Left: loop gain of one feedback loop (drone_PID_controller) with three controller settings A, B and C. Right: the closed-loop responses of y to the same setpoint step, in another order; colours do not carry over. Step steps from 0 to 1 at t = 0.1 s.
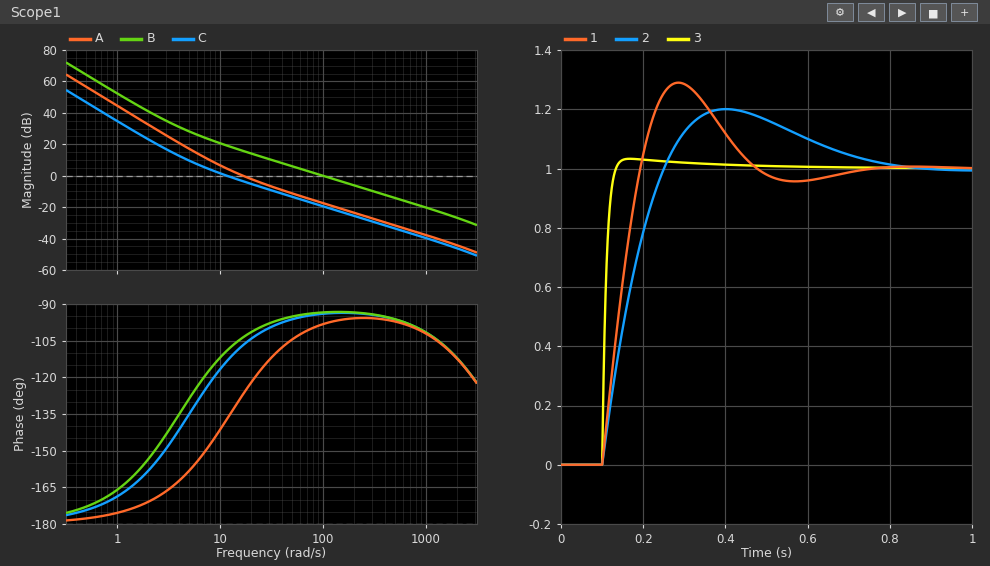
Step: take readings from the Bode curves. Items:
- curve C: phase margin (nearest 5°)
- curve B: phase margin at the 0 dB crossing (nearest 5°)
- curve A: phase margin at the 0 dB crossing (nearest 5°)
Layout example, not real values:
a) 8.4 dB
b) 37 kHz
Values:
a) 65°
b) 85°
c) 55°
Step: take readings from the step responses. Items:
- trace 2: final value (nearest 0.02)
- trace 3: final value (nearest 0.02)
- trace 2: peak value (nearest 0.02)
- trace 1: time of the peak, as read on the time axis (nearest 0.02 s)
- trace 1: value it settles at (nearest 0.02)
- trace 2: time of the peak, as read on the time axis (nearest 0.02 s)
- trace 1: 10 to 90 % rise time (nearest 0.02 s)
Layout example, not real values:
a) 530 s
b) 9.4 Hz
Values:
a) 1.00
b) 1.00
c) 1.20
d) 0.28 s
e) 1.00
f) 0.40 s
g) 0.08 s
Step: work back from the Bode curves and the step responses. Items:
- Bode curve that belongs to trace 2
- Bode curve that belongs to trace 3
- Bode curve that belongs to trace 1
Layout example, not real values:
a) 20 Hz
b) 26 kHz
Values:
a) C
b) B
c) A
